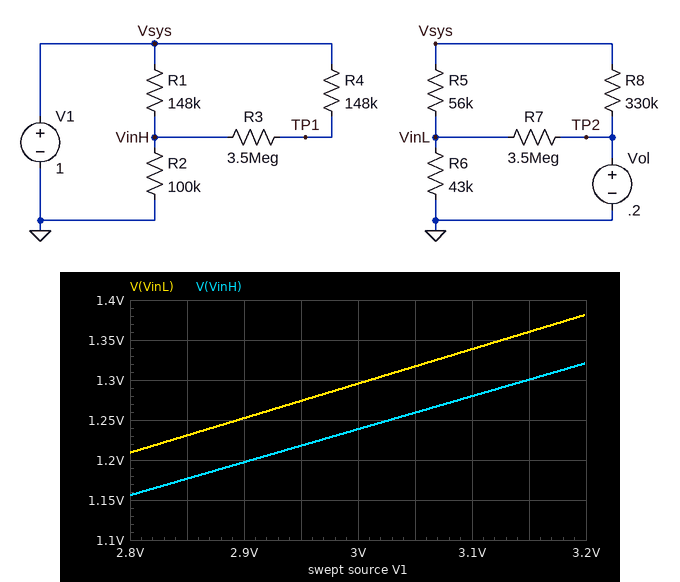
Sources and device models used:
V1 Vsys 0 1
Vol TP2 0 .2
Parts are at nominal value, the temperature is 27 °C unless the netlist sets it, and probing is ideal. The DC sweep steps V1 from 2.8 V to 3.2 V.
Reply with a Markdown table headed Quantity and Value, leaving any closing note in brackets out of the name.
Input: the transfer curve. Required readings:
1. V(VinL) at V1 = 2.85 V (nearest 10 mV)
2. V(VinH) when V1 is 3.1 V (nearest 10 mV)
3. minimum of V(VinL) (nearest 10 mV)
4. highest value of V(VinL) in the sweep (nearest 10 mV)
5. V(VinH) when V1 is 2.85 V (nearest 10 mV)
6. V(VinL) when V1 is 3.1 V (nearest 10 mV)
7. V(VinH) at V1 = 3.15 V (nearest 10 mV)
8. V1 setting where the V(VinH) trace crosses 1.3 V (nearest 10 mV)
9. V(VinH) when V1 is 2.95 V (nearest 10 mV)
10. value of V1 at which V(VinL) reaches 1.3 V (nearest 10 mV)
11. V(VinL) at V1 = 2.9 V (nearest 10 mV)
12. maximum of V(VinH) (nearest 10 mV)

| Quantity | Value |
|---|---|
| V(VinL) at V1 = 2.85 V | 1.23 V |
| V(VinH) when V1 is 3.1 V | 1.28 V |
| minimum of V(VinL) | 1.21 V |
| highest value of V(VinL) in the sweep | 1.38 V |
| V(VinH) when V1 is 2.85 V | 1.18 V |
| V(VinL) when V1 is 3.1 V | 1.34 V |
| V(VinH) at V1 = 3.15 V | 1.30 V |
| V1 setting where the V(VinH) trace crosses 1.3 V | 3.15 V |
| V(VinH) when V1 is 2.95 V | 1.22 V |
| value of V1 at which V(VinL) reaches 1.3 V | 3.01 V |
| V(VinL) at V1 = 2.9 V | 1.25 V |
| maximum of V(VinH) | 1.32 V |
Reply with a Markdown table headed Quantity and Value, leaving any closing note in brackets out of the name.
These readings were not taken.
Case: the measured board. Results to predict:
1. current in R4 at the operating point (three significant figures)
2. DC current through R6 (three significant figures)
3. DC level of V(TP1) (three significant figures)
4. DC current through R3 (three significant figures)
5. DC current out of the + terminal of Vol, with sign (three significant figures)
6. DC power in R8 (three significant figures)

| Quantity | Value |
|---|---|
| current in R4 at the operating point | 161 nA |
| DC current through R6 | 10.1 µA |
| DC level of V(TP1) | 976 mV |
| DC current through R3 | 161 nA |
| DC current out of the + terminal of Vol, with sign | -2.49 µA |
| DC power in R8 | 1.94 µW |
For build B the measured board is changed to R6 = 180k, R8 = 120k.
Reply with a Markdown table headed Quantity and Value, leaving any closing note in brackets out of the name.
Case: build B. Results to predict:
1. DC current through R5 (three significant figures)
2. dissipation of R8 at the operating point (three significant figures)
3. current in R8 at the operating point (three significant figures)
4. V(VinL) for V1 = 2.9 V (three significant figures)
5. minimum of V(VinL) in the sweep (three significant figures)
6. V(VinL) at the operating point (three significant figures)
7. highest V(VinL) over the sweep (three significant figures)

| Quantity | Value |
|---|---|
| DC current through R5 | 4.36 µA |
| dissipation of R8 at the operating point | 5.33 µW |
| current in R8 at the operating point | 6.67 µA |
| V(VinL) for V1 = 2.9 V | 2.19 V |
| minimum of V(VinL) in the sweep | 2.11 V |
| V(VinL) at the operating point | 756 mV |
| highest V(VinL) over the sweep | 2.41 V |
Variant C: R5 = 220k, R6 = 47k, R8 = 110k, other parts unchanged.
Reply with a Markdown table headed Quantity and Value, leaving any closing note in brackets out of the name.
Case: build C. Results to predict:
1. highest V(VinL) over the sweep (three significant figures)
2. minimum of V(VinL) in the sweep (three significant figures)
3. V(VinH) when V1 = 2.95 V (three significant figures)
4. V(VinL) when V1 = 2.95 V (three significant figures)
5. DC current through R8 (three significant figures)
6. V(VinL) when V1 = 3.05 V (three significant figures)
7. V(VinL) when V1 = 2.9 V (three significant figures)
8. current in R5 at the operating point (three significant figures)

| Quantity | Value |
|---|---|
| highest V(VinL) over the sweep | 559 mV |
| minimum of V(VinL) in the sweep | 490 mV |
| V(VinH) when V1 = 2.95 V | 1.22 V |
| V(VinL) when V1 = 2.95 V | 516 mV |
| DC current through R8 | 7.27 µA |
| V(VinL) when V1 = 3.05 V | 533 mV |
| V(VinL) when V1 = 2.9 V | 507 mV |
| current in R5 at the operating point | 3.74 µA |
